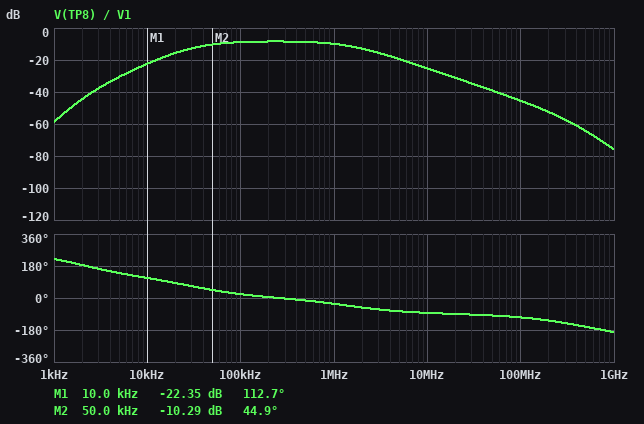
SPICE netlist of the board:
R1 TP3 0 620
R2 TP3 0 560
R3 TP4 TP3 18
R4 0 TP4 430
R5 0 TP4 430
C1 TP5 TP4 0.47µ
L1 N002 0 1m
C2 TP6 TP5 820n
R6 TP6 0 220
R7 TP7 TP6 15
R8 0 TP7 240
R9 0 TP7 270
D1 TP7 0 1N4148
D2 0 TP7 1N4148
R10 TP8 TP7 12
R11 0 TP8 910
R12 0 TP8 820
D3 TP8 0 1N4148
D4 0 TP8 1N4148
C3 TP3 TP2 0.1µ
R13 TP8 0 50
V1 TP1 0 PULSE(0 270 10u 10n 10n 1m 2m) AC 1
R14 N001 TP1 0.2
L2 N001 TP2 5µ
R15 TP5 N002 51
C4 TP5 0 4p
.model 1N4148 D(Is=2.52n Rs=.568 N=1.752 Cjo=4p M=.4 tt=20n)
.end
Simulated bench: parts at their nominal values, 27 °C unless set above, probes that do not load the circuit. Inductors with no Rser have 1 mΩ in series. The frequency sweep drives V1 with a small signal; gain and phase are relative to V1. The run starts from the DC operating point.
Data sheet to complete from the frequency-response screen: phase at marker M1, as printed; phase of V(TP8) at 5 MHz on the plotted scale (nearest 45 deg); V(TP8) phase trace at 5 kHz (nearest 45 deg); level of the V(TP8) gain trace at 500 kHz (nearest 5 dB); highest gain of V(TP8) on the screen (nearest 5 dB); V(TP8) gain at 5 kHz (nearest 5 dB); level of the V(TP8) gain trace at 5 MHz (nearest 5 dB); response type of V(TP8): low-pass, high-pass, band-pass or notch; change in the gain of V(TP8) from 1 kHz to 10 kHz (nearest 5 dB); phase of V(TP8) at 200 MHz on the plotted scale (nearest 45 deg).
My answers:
112.7 deg
-90 deg
135 deg
-10 dB
-10 dB
-30 dB
-20 dB
band-pass
35 dB
-135 deg
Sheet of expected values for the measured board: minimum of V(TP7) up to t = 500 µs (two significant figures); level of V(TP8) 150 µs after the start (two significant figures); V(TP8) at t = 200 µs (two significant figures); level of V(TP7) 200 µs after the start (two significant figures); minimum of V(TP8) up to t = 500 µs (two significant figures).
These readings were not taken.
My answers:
-1.1 V
190 mV
240 mV
310 mV
-710 mV
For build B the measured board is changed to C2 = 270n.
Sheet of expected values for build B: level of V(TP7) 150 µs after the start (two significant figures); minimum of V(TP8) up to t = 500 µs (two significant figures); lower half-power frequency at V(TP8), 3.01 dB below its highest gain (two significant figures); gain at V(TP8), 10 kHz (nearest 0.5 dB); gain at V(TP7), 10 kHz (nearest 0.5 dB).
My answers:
220 mV
-730 mV
42 kHz
-23.0 dB
-21.0 dB
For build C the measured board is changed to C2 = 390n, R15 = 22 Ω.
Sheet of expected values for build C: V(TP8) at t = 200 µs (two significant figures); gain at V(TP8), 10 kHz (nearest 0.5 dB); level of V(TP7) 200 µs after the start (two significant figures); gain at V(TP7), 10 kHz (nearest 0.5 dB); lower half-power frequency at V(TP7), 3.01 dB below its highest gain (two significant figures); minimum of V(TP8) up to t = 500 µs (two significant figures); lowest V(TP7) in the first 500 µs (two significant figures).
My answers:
-170 mV
-21.0 dB
-220 mV
-19.0 dB
39 kHz
-730 mV
-1.2 V
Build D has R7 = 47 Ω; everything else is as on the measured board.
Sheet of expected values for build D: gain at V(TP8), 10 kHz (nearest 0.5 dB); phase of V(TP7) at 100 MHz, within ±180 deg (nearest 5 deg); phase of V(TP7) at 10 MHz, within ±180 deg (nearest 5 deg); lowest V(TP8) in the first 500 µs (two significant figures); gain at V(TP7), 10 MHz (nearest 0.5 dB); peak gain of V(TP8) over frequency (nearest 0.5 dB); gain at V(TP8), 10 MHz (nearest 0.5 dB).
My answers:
-24.5 dB
-110 deg
-80 deg
-700 mV
-25.0 dB
-11.5 dB
-27.0 dB
